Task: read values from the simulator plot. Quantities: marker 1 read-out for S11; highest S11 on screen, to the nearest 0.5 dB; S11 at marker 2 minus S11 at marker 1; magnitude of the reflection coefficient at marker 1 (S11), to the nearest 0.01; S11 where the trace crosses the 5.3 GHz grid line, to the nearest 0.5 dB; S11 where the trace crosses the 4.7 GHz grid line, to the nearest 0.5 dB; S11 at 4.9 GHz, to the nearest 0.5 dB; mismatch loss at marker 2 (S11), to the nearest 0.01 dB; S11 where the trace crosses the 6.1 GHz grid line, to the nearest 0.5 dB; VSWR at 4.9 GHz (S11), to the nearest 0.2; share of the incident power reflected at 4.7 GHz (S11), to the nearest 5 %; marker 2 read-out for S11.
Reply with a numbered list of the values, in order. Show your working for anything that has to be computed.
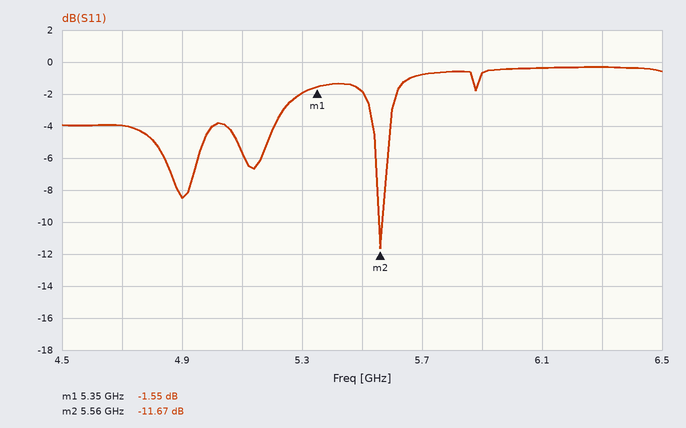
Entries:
1. -1.55 dB
2. -0.5 dB
3. -11.67 − (-1.55) = -10.12 dB
4. 10^(-1.55/20) ≈ 0.84
5. -2.0 dB
6. -4.0 dB
7. -8.5 dB
8. −10 log10(1 − 10^(-11.67/10)) ≈ 0.31 dB
9. -0.5 dB
10. |Γ| = 10^(-8.5/20) = 0.3758; VSWR = (1 + 0.3758)/(1 − 0.3758) ≈ 2.2
11. 10^(-4/10) ≈ 40 %
12. -11.67 dB
